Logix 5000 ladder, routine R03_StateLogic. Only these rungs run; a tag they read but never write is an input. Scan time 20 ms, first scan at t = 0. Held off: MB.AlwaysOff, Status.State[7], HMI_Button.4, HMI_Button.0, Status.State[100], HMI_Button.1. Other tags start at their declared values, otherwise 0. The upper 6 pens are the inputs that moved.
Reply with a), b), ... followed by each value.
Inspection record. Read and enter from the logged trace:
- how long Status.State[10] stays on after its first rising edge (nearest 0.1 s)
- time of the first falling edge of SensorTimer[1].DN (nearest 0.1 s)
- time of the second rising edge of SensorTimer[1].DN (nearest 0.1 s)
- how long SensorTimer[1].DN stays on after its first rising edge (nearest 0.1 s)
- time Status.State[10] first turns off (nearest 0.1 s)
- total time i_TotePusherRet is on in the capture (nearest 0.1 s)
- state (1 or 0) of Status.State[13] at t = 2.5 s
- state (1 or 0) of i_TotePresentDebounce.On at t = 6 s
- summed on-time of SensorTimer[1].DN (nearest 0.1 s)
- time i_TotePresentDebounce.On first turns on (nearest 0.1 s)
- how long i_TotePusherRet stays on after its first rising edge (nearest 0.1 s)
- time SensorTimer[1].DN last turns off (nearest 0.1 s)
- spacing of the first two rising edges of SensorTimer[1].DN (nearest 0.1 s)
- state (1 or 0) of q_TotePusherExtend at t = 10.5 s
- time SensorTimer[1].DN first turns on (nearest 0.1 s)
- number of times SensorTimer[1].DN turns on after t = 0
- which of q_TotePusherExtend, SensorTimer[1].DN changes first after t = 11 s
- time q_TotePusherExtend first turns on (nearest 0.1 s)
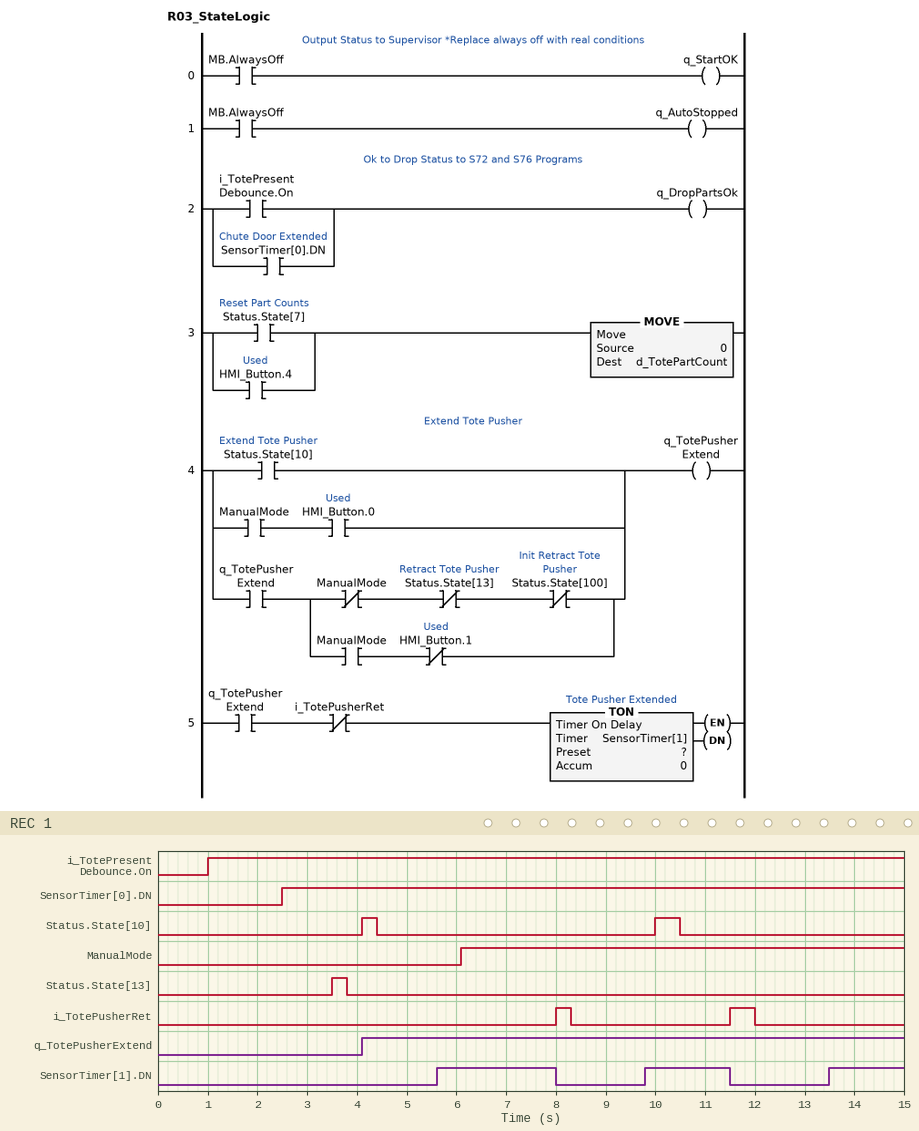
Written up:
a) 0.3 s
b) 8.0 s
c) 9.8 s
d) 2.4 s
e) 4.4 s
f) 0.8 s
g) 0
h) 1
i) 5.6 s
j) 1.0 s
k) 0.3 s
l) 11.5 s
m) 4.2 s
n) 1
o) 5.6 s
p) 3
q) SensorTimer[1].DN
r) 4.1 s
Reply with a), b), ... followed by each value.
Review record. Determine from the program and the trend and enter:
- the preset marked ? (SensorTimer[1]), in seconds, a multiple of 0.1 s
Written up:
a) 1.5 s
